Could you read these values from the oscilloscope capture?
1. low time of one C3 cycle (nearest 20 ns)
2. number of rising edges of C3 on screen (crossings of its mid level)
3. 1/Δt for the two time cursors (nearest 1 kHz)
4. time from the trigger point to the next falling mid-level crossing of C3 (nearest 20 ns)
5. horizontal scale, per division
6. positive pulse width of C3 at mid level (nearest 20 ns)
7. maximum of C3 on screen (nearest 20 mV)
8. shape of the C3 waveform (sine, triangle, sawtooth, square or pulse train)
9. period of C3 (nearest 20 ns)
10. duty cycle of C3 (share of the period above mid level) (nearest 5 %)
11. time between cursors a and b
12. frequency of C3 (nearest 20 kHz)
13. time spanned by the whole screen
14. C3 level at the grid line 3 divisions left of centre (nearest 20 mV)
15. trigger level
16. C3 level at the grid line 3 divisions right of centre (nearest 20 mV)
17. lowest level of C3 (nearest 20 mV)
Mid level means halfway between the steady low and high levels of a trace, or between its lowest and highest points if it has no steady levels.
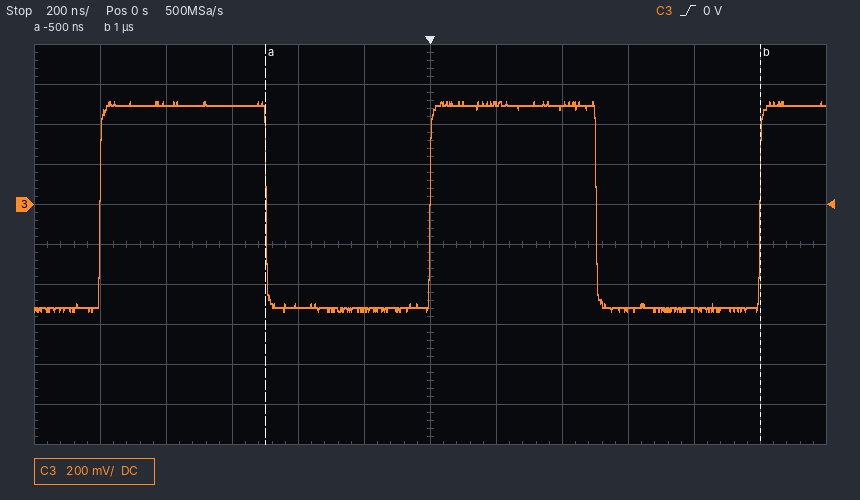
500 ns
3
667 kHz
500 ns
200 ns
500 ns
520 mV
square
1.00 µs
50 %
1.50 µs
1.00 MHz
2.4 µs
500 mV
0 V
-520 mV
-540 mV
